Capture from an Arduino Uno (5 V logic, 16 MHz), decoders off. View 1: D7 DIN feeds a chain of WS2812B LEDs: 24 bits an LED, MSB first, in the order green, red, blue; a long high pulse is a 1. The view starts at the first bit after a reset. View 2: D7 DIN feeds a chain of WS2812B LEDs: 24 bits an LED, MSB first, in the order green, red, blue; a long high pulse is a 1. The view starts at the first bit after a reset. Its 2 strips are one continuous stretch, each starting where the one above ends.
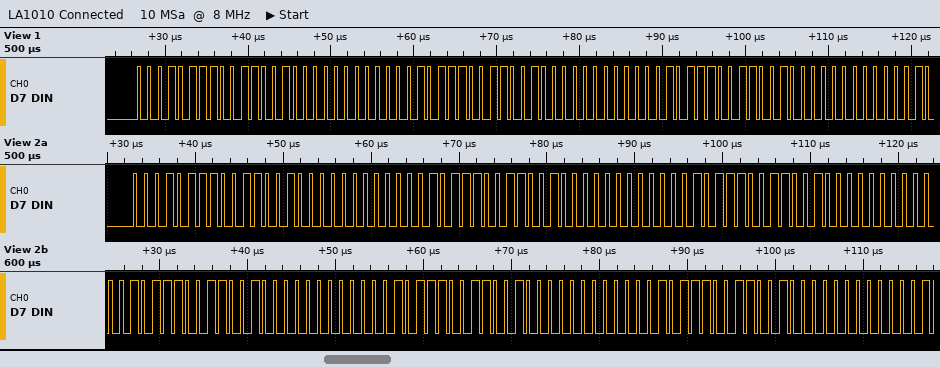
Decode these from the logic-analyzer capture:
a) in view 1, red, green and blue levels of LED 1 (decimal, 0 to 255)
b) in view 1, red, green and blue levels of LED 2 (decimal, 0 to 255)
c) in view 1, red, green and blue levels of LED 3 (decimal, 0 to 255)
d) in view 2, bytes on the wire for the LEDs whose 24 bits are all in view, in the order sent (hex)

50, 23, 0
50, 23, 0
50, 23, 0
17 32 00 17 32 00 17 32 00 17 32 00 17 32 00 17 32 00
